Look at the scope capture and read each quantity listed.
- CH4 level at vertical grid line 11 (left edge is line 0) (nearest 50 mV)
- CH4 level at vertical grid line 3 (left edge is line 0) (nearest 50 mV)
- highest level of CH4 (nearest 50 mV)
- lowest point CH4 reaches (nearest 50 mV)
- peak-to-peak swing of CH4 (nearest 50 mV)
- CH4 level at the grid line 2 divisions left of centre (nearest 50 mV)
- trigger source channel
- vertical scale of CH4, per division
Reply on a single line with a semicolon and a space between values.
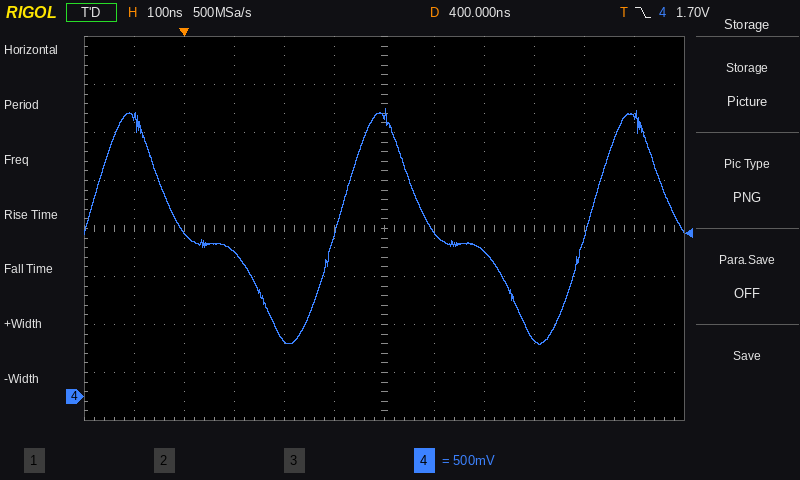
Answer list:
2.95 V; 1.50 V; 3.00 V; 550 mV; 2.45 V; 600 mV; CH4; 500 mV
